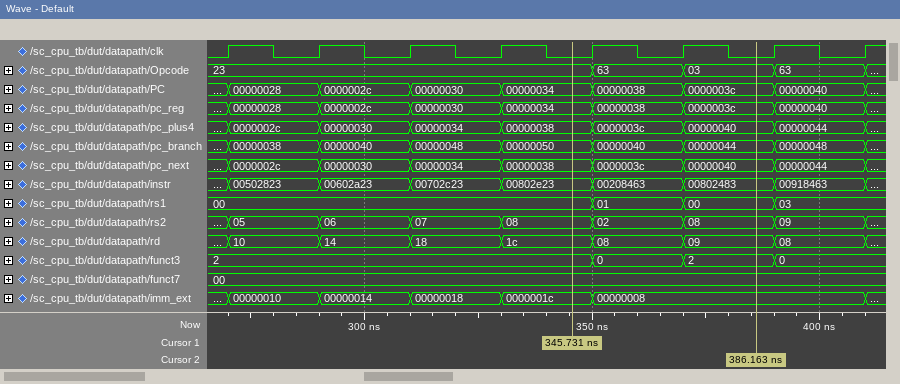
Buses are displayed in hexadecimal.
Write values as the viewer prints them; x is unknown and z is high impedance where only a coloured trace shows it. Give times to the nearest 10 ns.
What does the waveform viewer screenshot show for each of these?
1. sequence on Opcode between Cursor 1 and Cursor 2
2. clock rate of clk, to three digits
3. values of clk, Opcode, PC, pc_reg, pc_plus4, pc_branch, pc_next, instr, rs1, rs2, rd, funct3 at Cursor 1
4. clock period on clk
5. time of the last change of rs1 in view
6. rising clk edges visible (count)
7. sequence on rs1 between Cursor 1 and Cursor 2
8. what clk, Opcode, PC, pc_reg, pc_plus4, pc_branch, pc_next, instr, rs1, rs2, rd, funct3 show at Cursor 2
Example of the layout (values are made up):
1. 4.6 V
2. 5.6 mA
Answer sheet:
1. 23, 63, 03
2. 50.0 MHz
3. clk=0, Opcode=23, PC=00000034, pc_reg=00000034, pc_plus4=00000038, pc_branch=00000050, pc_next=00000038, instr=00802e23, rs1=00, rs2=08, rd=1c, funct3=2
4. 20 ns
5. 390 ns
6. 8
7. 00, 01, 00
8. clk=0, Opcode=03, PC=0000003c, pc_reg=0000003c, pc_plus4=00000040, pc_branch=00000044, pc_next=00000040, instr=00802483, rs1=00, rs2=08, rd=09, funct3=2
